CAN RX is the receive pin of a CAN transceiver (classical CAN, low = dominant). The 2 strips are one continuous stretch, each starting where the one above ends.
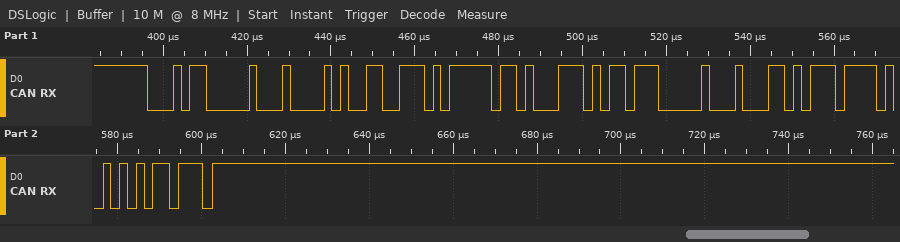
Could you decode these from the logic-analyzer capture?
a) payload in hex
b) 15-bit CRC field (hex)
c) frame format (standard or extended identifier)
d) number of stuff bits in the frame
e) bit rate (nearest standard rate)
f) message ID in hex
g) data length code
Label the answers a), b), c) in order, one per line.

a) 53 3A FE 8E B7 00 8D 77
b) 0x555B
c) standard
d) 3
e) 500 kbit/s
f) 0x160
g) 8
